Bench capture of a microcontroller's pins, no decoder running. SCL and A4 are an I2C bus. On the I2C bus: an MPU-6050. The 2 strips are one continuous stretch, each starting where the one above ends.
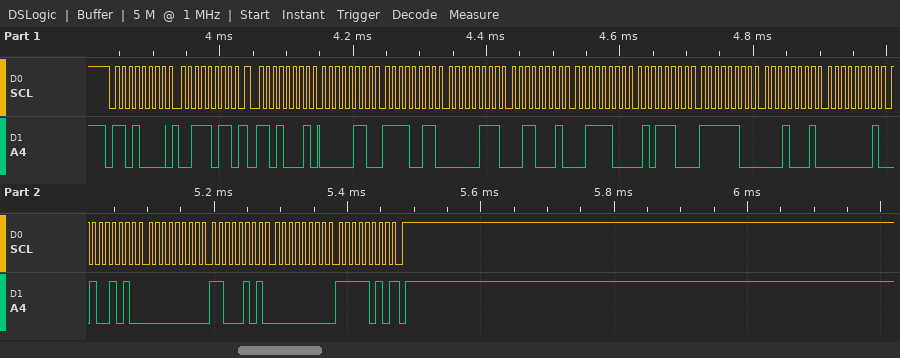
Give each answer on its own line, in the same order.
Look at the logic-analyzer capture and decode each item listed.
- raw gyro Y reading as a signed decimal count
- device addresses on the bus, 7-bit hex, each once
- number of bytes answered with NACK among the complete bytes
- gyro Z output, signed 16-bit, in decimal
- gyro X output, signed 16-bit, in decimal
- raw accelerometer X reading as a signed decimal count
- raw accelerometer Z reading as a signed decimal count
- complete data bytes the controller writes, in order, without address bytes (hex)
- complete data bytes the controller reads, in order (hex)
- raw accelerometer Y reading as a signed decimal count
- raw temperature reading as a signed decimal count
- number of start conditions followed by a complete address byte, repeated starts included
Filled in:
197
0x68
1
250
330
1779
15452
3B
06 F3 07 31 3C 5C FC 11 01 4A 00 C5 00 FA
1841
-1007
2
